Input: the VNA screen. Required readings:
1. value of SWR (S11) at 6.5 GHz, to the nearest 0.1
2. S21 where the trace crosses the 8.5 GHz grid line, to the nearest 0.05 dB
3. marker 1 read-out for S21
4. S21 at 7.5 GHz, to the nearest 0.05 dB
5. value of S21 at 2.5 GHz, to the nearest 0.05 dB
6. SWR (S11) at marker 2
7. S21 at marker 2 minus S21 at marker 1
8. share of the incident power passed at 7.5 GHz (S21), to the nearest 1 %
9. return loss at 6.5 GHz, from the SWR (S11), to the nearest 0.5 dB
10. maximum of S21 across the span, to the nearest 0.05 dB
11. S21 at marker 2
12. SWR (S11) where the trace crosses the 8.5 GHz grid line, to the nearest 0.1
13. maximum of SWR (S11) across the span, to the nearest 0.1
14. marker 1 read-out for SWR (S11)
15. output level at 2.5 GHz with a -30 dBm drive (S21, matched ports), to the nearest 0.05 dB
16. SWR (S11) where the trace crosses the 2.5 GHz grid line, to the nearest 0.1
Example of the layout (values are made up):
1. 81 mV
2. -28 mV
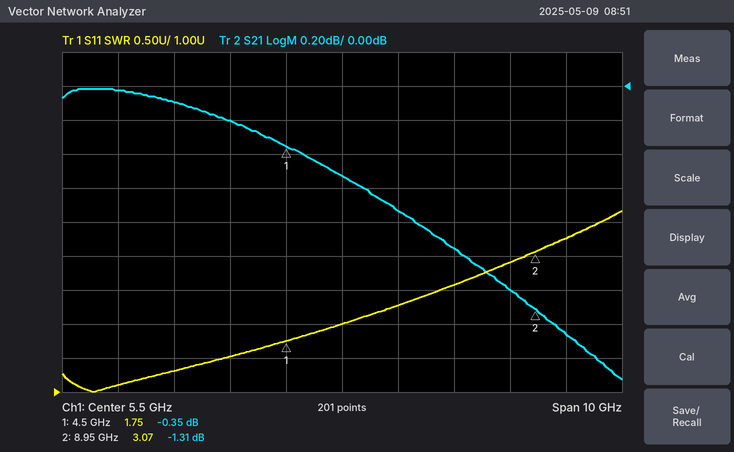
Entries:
1. 2.3
2. -1.20 dB
3. -0.35 dB
4. -0.95 dB
5. -0.10 dB
6. 3.07
7. -0.96 dB
8. 80 %
9. 8.0 dB
10. 0.00 dB
11. -1.31 dB
12. 2.9
13. 3.7
14. 1.75
15. -30.10 dBm
16. 1.3
